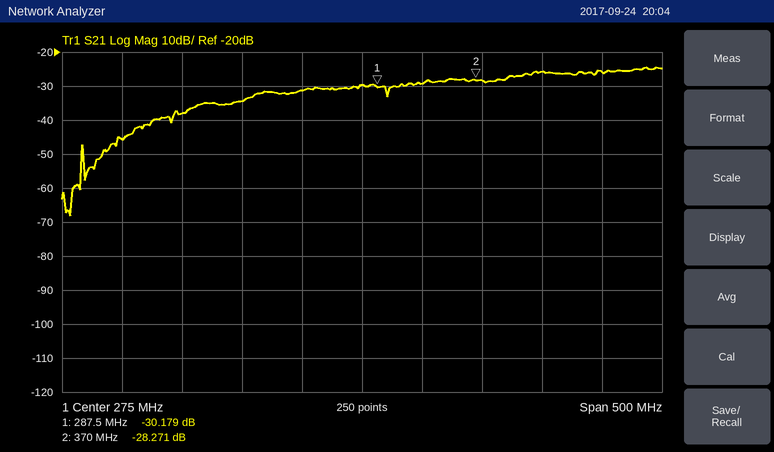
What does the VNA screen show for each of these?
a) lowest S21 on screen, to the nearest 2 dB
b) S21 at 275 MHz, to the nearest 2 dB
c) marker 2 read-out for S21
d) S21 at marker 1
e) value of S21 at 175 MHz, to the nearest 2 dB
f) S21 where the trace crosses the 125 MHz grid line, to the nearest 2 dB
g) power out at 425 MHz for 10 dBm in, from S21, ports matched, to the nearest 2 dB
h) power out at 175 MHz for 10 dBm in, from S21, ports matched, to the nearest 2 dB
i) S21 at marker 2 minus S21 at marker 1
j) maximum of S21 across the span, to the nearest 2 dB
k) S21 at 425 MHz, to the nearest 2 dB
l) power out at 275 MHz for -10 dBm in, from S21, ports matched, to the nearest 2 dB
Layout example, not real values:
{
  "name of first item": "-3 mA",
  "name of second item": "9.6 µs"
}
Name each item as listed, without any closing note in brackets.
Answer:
{
  "lowest S21 on screen, to the nearest 2 dB": "-68 dB",
  "S21 at 275 MHz, to the nearest 2 dB": "-30 dB",
  "marker 2 read-out for S21": "-28.271 dB",
  "S21 at marker 1": "-30.179 dB",
  "value of S21 at 175 MHz, to the nearest 2 dB": "-34 dB",
  "S21 where the trace crosses the 125 MHz grid line, to the nearest 2 dB": "-38 dB",
  "power out at 425 MHz for 10 dBm in, from S21, ports matched, to the nearest 2 dB": "-16 dBm",
  "power out at 175 MHz for 10 dBm in, from S21, ports matched, to the nearest 2 dB": "-24 dBm",
  "S21 at marker 2 minus S21 at marker 1": "1.908 dB",
  "maximum of S21 across the span, to the nearest 2 dB": "-24 dB",
  "S21 at 425 MHz, to the nearest 2 dB": "-26 dB",
  "power out at 275 MHz for -10 dBm in, from S21, ports matched, to the nearest 2 dB": "-40 dBm"
}
